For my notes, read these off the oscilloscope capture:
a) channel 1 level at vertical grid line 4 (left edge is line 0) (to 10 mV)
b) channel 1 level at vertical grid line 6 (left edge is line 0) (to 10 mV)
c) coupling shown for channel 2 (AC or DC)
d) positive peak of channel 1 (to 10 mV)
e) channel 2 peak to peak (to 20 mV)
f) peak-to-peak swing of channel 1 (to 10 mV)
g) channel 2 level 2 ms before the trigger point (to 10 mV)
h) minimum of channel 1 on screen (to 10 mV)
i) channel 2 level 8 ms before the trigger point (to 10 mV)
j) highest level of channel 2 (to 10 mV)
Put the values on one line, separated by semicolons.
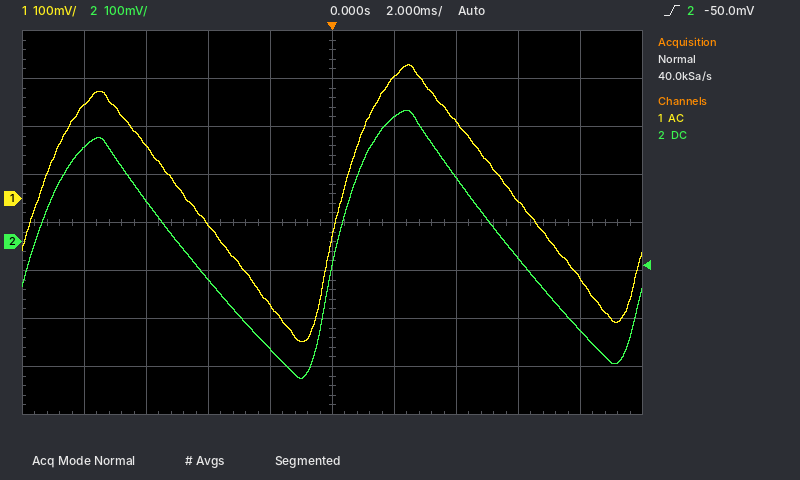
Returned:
-220 mV; 250 mV; DC; 280 mV; 560 mV; 580 mV; -220 mV; -300 mV; 200 mV; 270 mV
